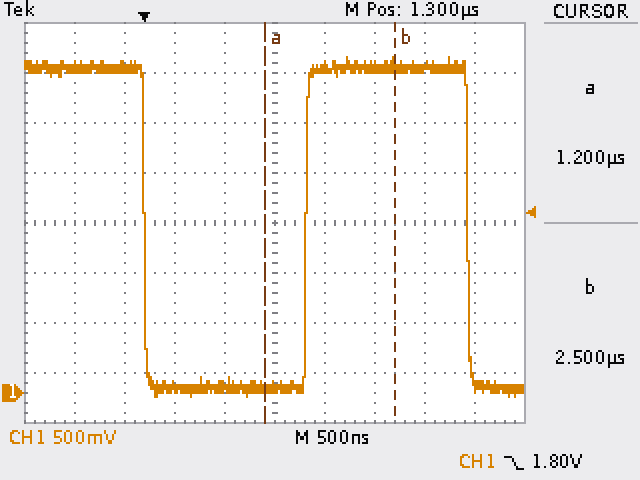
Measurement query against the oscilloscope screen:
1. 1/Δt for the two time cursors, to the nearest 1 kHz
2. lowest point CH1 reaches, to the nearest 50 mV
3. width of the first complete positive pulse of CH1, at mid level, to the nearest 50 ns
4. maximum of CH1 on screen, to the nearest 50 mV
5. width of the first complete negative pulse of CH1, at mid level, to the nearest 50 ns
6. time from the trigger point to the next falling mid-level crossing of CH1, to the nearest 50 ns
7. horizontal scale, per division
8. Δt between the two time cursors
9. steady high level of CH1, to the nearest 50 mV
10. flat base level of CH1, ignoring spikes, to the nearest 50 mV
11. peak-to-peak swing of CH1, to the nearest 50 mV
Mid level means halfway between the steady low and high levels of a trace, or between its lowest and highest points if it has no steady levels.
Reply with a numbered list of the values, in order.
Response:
1. 769 kHz
2. -50 mV
3. 1.60 µs
4. 3.35 V
5. 1.60 µs
6. 3.25 µs
7. 500 ns
8. 1.30 µs
9. 3.25 V
10. 50 mV
11. 3.40 V
